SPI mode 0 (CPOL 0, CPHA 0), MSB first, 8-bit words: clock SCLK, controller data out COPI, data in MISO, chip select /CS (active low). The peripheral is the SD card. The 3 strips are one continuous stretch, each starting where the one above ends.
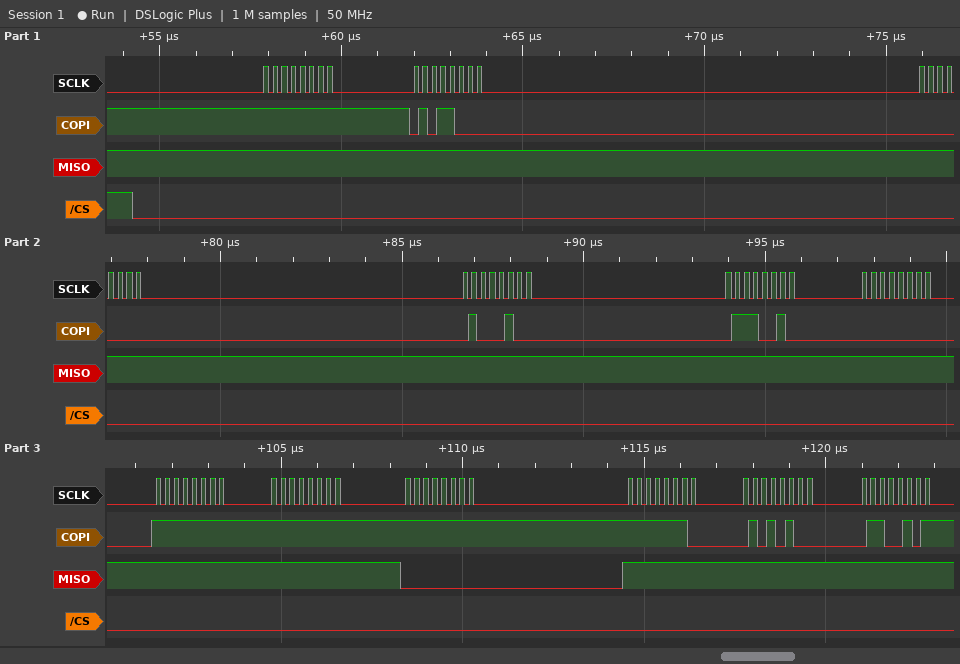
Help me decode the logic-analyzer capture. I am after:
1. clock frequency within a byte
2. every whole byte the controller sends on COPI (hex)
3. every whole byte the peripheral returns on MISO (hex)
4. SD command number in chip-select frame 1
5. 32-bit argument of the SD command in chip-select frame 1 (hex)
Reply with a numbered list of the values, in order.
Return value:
1. 4 MHz
2. FF 58 00 44 72 00 FF FF FF FE 54 65
3. FF FF FF FF FF FF FF FF 00 FF FF FF
4. CMD24
5. 0x00447200
